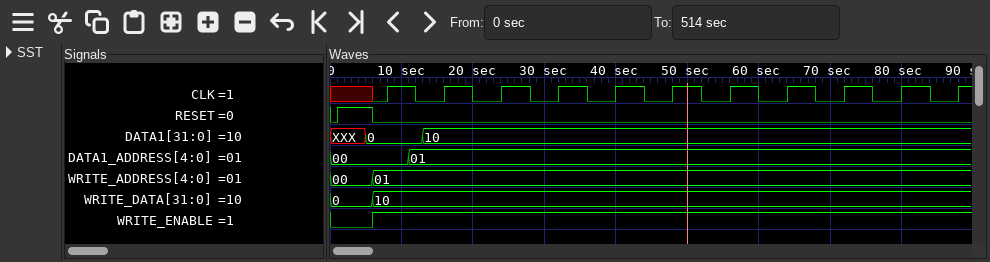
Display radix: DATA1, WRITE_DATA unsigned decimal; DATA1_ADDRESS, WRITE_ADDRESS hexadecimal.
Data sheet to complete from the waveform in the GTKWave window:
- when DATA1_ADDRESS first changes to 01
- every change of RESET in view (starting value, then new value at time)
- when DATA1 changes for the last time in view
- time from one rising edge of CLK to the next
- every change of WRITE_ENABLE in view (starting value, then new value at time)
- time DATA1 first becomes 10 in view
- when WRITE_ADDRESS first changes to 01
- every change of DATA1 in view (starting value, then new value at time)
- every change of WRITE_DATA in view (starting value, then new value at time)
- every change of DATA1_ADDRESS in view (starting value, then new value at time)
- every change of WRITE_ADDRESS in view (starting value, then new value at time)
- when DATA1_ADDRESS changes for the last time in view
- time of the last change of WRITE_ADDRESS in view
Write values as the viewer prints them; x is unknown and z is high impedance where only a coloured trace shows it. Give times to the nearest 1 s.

11 s
0, 1 at 1 s, 0 at 6 s
13 s
8 s
0, 1 at 6 s
13 s
6 s
XXX, 0 at 5 s, 10 at 13 s
0, 10 at 6 s
00, 01 at 11 s
00, 01 at 6 s
11 s
6 s
